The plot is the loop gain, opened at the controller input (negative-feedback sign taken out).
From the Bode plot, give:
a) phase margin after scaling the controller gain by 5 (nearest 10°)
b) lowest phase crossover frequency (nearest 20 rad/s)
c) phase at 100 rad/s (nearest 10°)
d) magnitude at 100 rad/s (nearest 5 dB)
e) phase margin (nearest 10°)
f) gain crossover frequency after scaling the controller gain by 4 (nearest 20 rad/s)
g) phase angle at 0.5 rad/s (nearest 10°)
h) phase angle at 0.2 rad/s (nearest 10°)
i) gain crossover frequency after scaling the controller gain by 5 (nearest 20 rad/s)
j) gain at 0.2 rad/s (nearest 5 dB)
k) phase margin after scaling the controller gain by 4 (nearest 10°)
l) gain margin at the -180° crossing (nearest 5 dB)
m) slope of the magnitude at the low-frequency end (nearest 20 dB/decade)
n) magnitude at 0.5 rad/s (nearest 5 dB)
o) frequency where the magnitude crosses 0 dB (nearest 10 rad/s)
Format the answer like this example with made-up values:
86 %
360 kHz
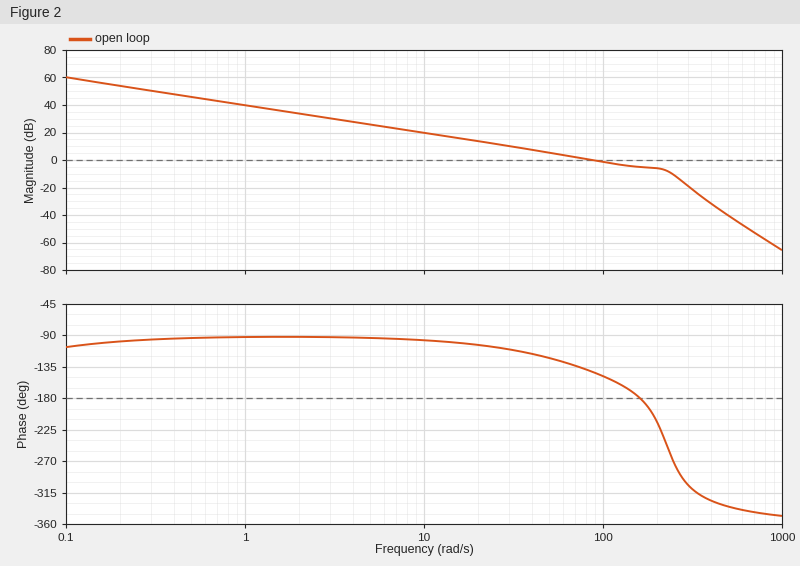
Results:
-110°
160 rad/s
-150°
0 dB
40°
260 rad/s
-90°
-100°
260 rad/s
55 dB
-100°
5 dB
-20 dB/decade
45 dB
90 rad/s
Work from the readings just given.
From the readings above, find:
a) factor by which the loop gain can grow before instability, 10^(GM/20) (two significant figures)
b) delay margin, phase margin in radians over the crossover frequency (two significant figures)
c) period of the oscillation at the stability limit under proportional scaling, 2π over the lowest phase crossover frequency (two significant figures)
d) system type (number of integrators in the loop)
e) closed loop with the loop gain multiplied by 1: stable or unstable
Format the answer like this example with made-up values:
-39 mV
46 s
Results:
1.8
0.0078 s
0.039 s
1
stable
